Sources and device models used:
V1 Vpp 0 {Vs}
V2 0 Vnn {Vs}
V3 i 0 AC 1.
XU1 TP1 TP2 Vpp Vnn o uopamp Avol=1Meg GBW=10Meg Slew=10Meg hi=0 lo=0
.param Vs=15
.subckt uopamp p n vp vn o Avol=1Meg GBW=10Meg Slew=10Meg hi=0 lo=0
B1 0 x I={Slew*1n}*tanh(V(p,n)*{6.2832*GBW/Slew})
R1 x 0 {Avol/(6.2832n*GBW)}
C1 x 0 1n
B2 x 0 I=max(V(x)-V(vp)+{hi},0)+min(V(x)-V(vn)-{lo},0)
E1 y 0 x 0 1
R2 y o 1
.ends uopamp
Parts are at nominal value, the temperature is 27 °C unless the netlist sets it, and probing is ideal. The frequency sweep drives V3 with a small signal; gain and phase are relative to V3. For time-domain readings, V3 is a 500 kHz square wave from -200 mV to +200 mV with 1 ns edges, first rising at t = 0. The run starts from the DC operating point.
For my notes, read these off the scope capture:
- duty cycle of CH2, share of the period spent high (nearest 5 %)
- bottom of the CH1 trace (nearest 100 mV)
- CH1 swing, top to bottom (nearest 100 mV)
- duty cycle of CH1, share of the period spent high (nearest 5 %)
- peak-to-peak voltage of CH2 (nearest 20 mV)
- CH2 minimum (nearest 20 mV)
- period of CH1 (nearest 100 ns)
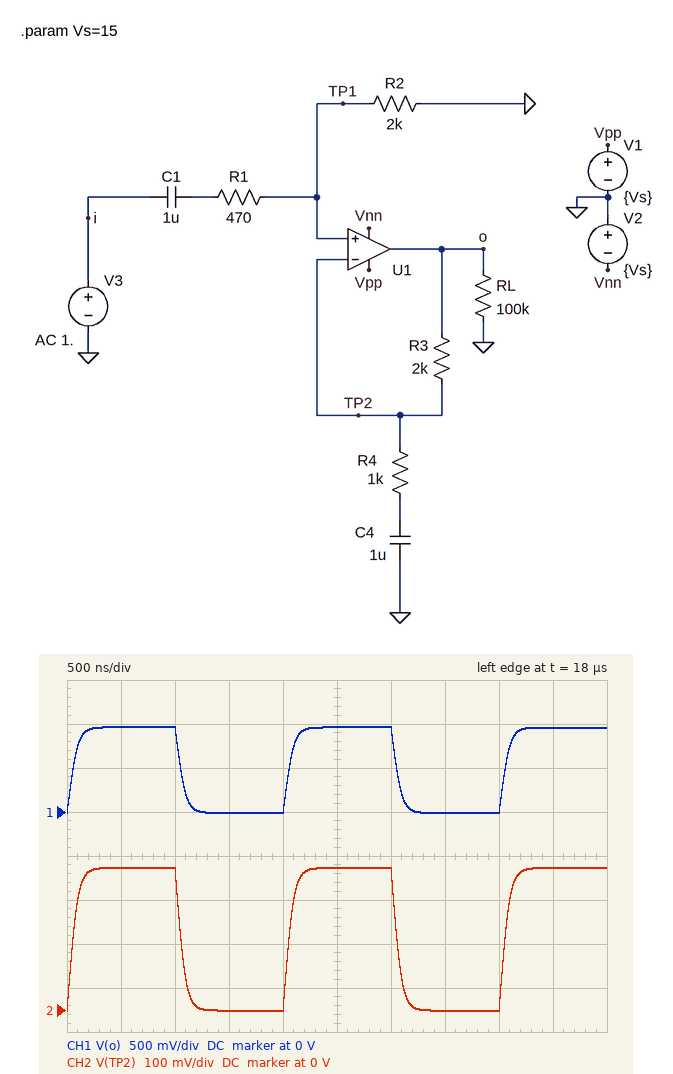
50 %
0 V
1.0 V
50 %
320 mV
0 V
2.0 µs
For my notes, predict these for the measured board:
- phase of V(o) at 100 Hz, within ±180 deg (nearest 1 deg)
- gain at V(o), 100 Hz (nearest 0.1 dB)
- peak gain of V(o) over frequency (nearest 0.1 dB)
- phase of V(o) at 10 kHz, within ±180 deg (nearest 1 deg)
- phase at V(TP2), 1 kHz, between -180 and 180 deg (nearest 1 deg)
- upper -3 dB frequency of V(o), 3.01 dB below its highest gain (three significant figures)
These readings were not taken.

63 deg
1.8 dB
7.7 dB
1 deg
4 deg
3.33 MHz
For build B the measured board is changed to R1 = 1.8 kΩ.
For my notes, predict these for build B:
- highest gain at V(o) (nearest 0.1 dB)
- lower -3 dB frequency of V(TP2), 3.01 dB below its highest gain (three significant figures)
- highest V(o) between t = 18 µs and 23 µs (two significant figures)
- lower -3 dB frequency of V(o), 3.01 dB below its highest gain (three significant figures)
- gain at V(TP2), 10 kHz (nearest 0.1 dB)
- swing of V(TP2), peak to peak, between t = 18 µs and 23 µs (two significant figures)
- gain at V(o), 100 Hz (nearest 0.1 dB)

4.0 dB
41.9 Hz
630 mV
153 Hz
-5.6 dB
210 mV
-1.1 dB
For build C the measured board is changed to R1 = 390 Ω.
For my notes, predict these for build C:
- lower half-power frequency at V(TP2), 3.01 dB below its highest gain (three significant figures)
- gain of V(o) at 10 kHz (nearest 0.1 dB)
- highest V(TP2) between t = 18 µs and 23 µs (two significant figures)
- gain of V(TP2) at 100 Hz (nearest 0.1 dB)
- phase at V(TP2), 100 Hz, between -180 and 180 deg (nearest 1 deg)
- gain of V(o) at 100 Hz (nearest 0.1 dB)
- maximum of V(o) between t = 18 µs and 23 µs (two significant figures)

66.6 Hz
8.0 dB
330 mV
-3.1 dB
34 deg
2.0 dB
990 mV
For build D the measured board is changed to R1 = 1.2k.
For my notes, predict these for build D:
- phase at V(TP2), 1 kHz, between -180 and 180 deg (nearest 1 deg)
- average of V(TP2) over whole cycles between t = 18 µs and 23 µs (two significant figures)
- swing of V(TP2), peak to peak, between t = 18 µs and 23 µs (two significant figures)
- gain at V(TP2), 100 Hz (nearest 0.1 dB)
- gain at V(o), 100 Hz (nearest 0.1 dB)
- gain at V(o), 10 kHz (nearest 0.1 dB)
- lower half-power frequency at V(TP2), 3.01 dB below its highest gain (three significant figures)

3 deg
120 mV
250 mV
-5.0 dB
0.1 dB
5.5 dB
49.7 Hz
